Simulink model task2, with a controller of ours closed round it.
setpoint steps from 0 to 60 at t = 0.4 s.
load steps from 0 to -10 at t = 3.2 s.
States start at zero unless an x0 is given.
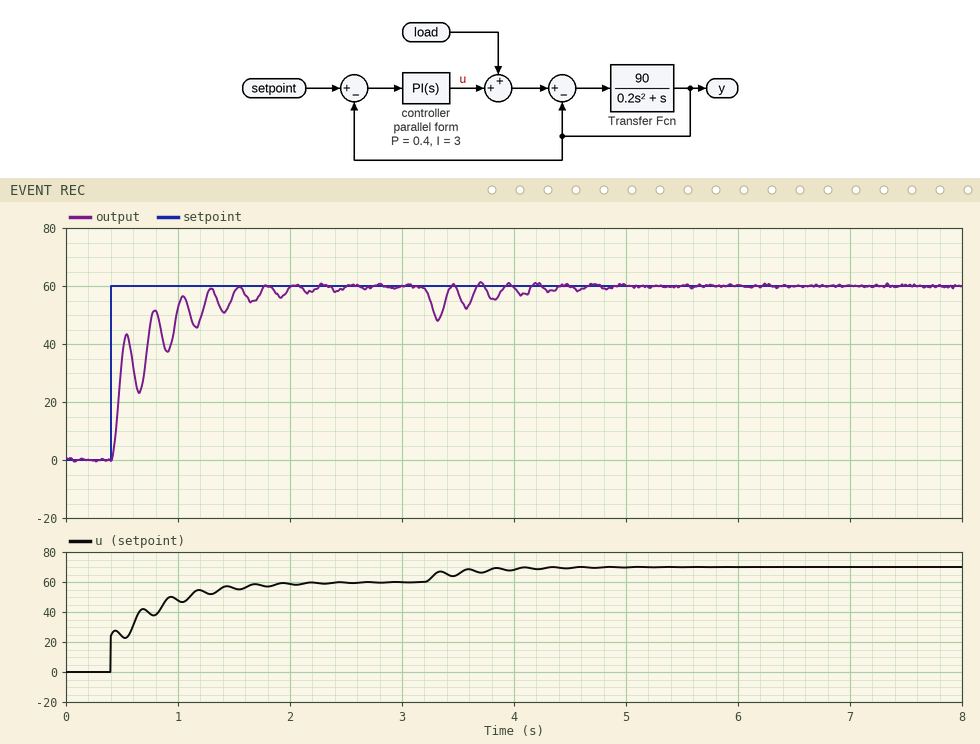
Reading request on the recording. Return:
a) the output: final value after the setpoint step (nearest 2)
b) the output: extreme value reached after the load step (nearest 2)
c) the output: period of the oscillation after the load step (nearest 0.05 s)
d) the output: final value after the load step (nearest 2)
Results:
60
48
0.25 s
60
